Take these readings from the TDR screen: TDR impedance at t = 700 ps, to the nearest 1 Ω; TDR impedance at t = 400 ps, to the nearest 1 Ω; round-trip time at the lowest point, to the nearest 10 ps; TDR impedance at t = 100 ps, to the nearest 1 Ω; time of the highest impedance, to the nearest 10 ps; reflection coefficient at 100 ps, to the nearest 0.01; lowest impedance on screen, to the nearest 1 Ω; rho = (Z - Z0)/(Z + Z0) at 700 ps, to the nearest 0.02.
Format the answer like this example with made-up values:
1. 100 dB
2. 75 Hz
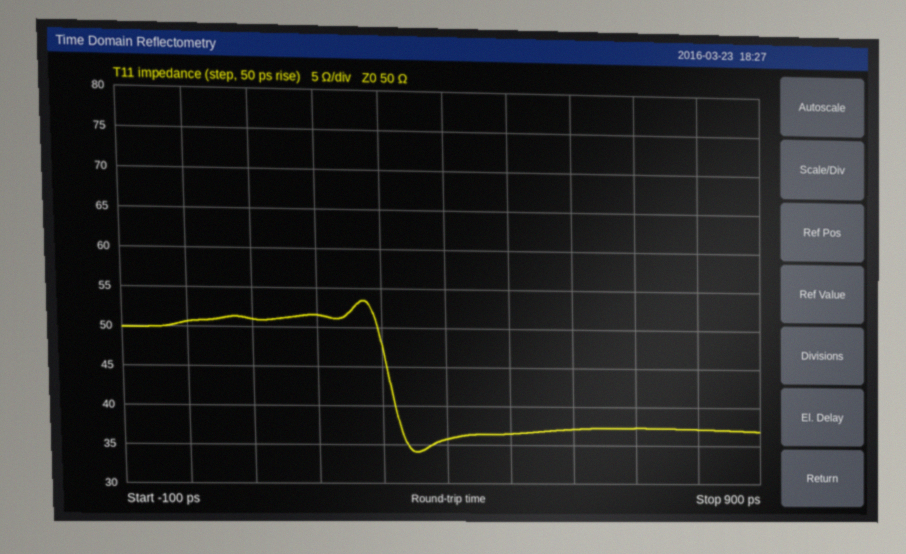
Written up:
1. 37 Ω
2. 36 Ω
3. 350 ps
4. 51 Ω
5. 270 ps
6. +0.01
7. 34 Ω
8. -0.14
